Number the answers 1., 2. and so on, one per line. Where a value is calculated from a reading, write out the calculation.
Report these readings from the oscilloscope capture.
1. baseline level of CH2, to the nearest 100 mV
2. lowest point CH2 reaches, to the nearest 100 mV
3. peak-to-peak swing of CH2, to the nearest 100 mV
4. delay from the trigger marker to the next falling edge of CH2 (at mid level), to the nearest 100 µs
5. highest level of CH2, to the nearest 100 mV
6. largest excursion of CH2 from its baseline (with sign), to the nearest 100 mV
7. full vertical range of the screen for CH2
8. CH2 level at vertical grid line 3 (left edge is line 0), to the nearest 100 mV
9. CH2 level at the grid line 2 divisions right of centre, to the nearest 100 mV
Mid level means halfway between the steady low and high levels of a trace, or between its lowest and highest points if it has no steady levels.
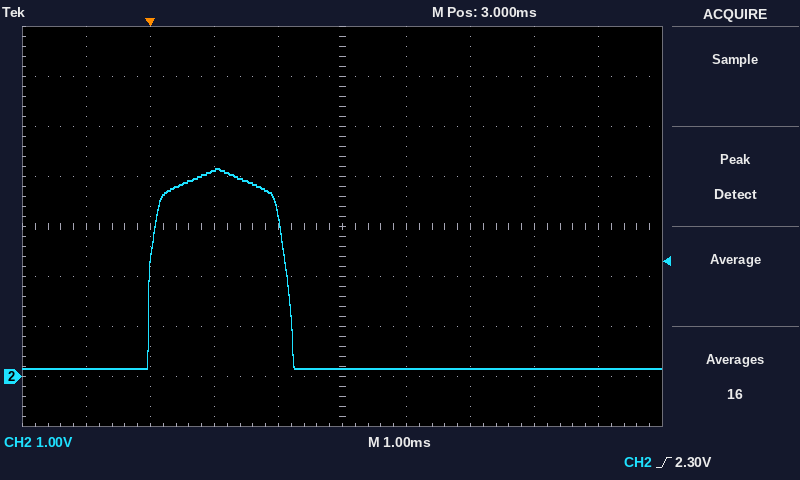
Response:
1. 200 mV
2. 200 mV
3. 4.2 V − (200 mV) = 4.0 V
4. 2.1 ms
5. 4.2 V
6. 4.2 V − (200 mV) = +4.0 V
7. 8 V
8. 4.1 V
9. 200 mV
